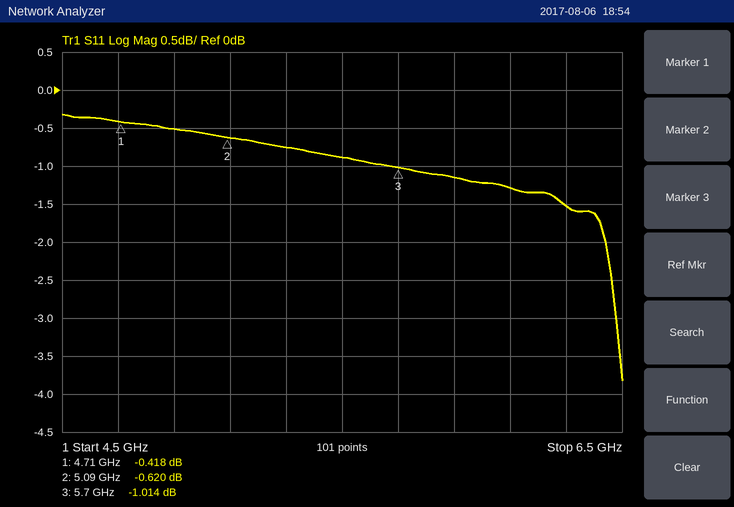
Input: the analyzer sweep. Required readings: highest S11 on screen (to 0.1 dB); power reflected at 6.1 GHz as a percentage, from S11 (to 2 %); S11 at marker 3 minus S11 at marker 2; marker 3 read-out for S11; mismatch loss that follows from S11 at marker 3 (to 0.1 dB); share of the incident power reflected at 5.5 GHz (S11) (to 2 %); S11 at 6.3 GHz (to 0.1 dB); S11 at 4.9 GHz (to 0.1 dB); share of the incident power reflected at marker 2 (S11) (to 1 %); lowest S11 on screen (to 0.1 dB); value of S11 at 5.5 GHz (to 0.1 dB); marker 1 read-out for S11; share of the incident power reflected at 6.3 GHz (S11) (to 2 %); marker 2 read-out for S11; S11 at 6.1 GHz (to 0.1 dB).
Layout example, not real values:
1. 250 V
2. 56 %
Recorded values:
1. -0.3 dB
2. 74 %
3. -0.394 dB
4. -1.014 dB
5. 6.8 dB
6. 82 %
7. -1.5 dB
8. -0.5 dB
9. 87 %
10. -3.8 dB
11. -0.9 dB
12. -0.418 dB
13. 70 %
14. -0.620 dB
15. -1.3 dB
